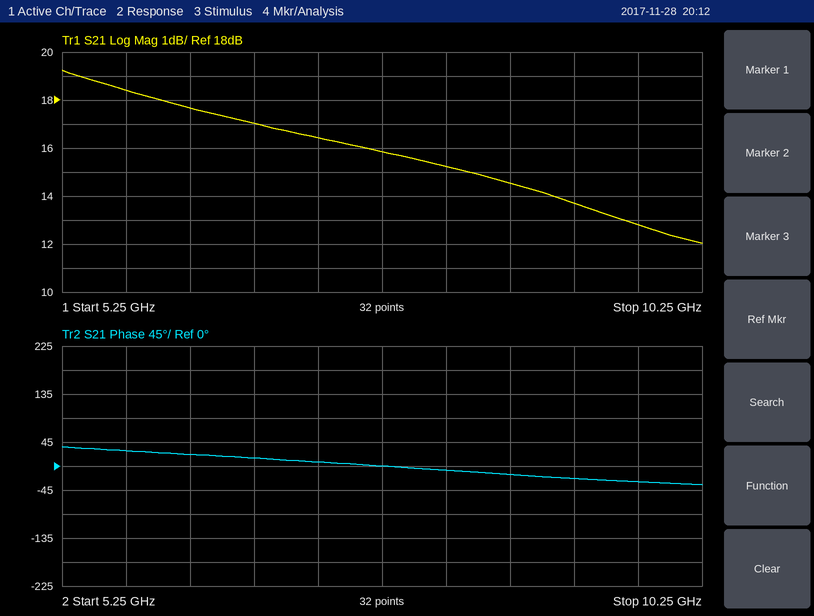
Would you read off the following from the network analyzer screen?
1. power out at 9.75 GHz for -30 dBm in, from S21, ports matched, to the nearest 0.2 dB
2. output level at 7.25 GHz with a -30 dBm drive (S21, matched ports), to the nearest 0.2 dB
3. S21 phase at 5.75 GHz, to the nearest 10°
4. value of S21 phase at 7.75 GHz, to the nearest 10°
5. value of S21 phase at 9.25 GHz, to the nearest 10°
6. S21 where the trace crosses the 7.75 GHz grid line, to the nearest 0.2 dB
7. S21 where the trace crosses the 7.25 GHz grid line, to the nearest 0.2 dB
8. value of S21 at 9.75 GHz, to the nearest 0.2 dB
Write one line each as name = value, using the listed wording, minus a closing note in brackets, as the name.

power out at 9.75 GHz for -30 dBm in, from S21, ports matched, to the nearest 0.2 dB = -17.2 dBm
output level at 7.25 GHz with a -30 dBm drive (S21, matched ports), to the nearest 0.2 dB = -13.6 dBm
S21 phase at 5.75 GHz, to the nearest 10° = 30°
value of S21 phase at 7.75 GHz, to the nearest 10° = 0°
value of S21 phase at 9.25 GHz, to the nearest 10° = -20°
S21 where the trace crosses the 7.75 GHz grid line, to the nearest 0.2 dB = 15.8 dB
S21 where the trace crosses the 7.25 GHz grid line, to the nearest 0.2 dB = 16.4 dB
value of S21 at 9.75 GHz, to the nearest 0.2 dB = 12.8 dB
